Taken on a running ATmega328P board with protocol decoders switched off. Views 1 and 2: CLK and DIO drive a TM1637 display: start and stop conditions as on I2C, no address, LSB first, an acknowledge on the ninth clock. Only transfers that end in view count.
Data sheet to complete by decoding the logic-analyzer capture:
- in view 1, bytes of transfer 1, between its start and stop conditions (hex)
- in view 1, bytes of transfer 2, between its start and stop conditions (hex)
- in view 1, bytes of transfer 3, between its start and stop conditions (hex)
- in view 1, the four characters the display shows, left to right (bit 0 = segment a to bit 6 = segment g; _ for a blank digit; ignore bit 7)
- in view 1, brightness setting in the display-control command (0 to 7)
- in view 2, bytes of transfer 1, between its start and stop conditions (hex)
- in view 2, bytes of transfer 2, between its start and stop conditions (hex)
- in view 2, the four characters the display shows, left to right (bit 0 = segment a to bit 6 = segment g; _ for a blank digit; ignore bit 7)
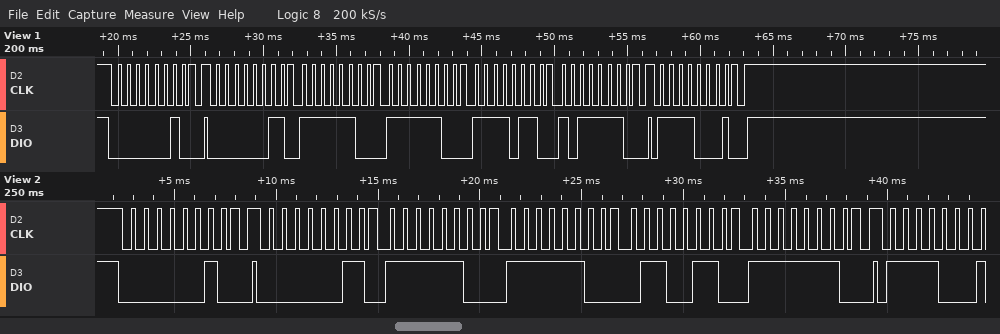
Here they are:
40
C0 3F 3F 6F 7D
8F
0096
7
40
C0 3F 3F 66 7F
0048
